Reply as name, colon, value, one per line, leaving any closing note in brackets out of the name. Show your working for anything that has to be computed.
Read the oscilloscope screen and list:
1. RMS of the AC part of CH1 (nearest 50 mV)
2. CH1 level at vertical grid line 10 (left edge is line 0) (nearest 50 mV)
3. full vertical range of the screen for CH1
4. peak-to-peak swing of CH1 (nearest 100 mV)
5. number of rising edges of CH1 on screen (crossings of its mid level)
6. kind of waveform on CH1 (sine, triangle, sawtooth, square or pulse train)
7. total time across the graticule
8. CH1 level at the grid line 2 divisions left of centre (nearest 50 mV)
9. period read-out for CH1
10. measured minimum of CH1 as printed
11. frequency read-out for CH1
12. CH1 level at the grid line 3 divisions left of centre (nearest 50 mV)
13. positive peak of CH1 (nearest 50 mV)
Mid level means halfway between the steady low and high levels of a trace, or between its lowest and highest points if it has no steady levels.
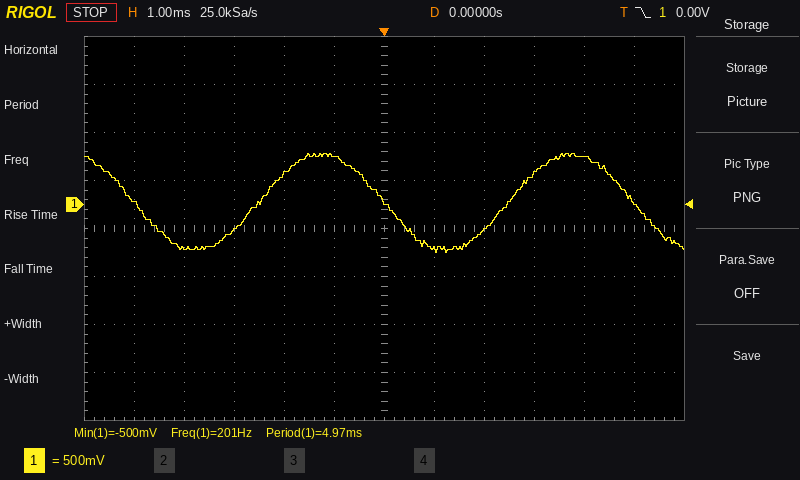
RMS of the AC part of CH1: 1.00 V / (2√2) ≈ 354 mV, so 350 mV to the nearest 50 mV
CH1 level at vertical grid line 10 (left edge is line 0): 500 mV
full vertical range of the screen for CH1: 4 V
peak-to-peak swing of CH1: 1.00 V
number of rising edges of CH1 on screen: 2
kind of waveform on CH1: sine
total time across the graticule: 12 ms
CH1 level at the grid line 2 divisions left of centre: 300 mV
period read-out for CH1: 4.97 ms
measured minimum of CH1 as printed: -500 mV
frequency read-out for CH1: 201 Hz
CH1 level at the grid line 3 divisions left of centre: -250 mV
positive peak of CH1: 550 mV
